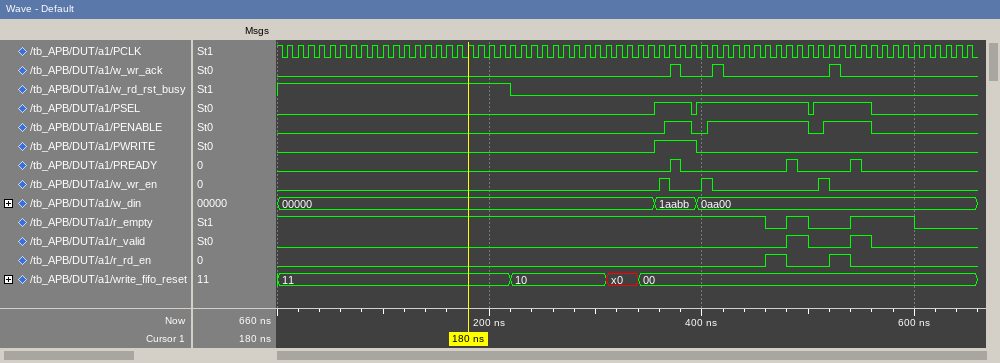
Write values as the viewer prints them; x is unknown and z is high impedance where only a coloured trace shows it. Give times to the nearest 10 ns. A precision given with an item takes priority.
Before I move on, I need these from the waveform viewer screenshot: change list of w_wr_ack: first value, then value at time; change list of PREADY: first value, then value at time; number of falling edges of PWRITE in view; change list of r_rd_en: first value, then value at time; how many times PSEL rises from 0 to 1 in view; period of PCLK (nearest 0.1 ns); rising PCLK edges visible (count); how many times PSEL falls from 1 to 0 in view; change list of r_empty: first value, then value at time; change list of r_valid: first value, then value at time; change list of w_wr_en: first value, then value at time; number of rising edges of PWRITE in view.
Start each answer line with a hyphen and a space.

- 0, 1 at 370 ns, 0 at 380 ns, 1 at 410 ns, 0 at 420 ns, 1 at 520 ns, 0 at 530 ns
- 0, 1 at 370 ns, 0 at 380 ns, 1 at 480 ns, 0 at 490 ns, 1 at 540 ns, 0 at 550 ns
- 1
- 0, 1 at 460 ns, 0 at 480 ns, 1 at 520 ns, 0 at 540 ns
- 3
- 10 ns
- 65
- 3
- 1, 0 at 460 ns, 1 at 480 ns, 0 at 500 ns, 1 at 540 ns, 0 at 600 ns
- 0, 1 at 480 ns, 0 at 500 ns, 1 at 540 ns, 0 at 560 ns
- 0, 1 at 360 ns, 0 at 370 ns, 1 at 400 ns, 0 at 410 ns, 1 at 510 ns, 0 at 520 ns
- 1
